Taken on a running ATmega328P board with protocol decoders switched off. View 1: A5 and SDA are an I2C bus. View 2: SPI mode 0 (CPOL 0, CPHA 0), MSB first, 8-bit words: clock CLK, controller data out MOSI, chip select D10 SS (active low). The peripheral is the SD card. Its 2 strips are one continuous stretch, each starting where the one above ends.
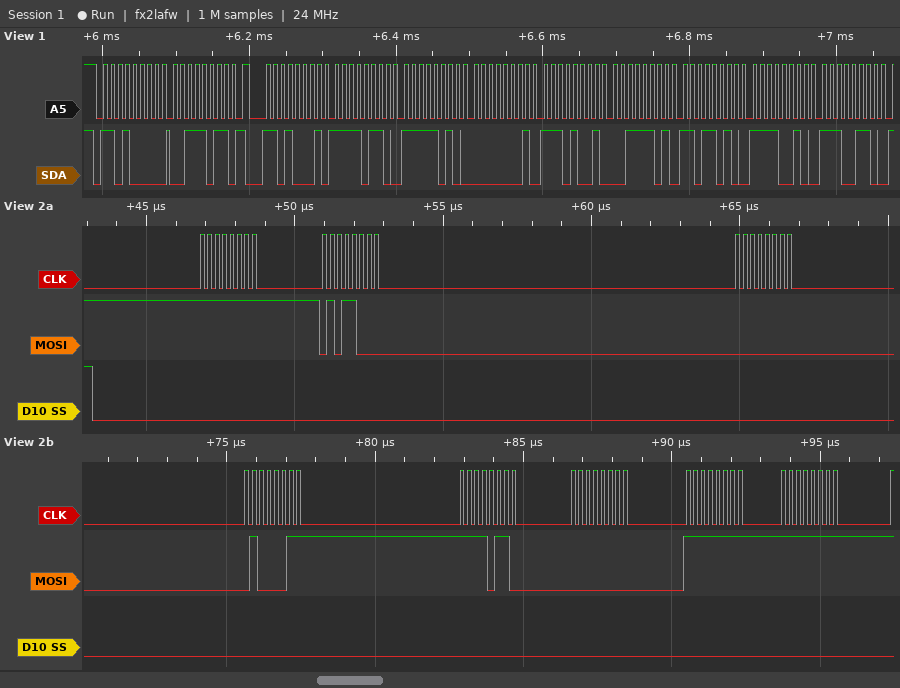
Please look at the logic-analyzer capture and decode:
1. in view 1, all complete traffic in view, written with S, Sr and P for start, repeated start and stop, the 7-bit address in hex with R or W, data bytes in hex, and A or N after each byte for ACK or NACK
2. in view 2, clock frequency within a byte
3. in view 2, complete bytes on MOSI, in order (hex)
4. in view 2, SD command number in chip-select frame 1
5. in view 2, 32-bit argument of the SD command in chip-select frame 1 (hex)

S 68W A 3B A Sr 68R A F6 A FA A 01 A E9 A 3D A DA A F2 A E6 A
4 MHz
0xFF 0x58 0x00 0x43 0xF6 0x00 0xFF 0xFF
CMD24
0x0043F600
